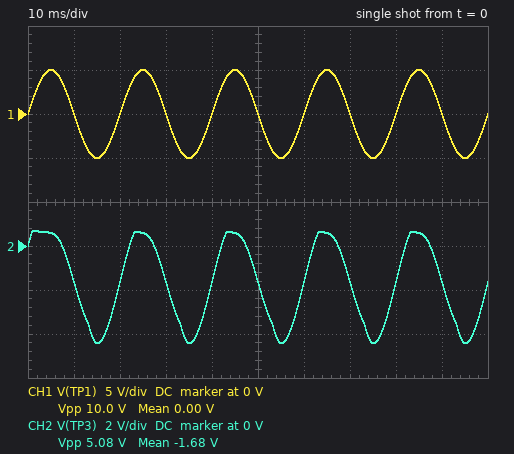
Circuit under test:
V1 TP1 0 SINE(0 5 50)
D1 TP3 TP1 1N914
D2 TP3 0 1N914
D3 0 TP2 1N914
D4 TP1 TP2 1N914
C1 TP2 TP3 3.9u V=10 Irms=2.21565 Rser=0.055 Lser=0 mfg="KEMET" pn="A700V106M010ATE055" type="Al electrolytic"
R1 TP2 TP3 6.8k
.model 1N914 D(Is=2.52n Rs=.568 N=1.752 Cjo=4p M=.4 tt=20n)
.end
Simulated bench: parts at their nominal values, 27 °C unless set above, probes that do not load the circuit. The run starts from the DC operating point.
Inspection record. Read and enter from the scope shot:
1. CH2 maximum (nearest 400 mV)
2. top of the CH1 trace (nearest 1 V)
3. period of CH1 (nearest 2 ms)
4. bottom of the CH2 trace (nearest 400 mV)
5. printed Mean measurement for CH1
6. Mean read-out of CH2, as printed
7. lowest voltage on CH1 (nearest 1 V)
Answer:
800 mV
5 V
20 ms
-4.4 V
0.00 V
-1.68 V
-5 V
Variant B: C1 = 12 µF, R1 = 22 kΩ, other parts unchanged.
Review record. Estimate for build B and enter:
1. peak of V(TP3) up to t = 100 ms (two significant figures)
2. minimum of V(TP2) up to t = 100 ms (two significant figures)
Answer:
720 mV
-610 mV
